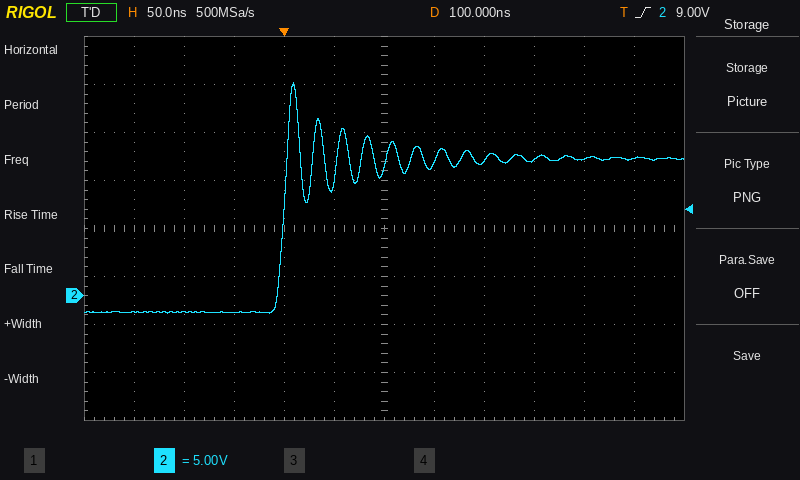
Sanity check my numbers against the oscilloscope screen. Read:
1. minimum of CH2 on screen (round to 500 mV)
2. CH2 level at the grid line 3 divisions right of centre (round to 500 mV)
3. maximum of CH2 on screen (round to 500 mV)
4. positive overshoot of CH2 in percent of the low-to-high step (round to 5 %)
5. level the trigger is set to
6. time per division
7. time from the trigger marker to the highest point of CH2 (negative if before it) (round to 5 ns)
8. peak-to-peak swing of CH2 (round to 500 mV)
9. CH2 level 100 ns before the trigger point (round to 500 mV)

-2.0 V
14.0 V
22.0 V
50 %
9.00 V
50 ns
+10 ns
24.0 V
-1.5 V
